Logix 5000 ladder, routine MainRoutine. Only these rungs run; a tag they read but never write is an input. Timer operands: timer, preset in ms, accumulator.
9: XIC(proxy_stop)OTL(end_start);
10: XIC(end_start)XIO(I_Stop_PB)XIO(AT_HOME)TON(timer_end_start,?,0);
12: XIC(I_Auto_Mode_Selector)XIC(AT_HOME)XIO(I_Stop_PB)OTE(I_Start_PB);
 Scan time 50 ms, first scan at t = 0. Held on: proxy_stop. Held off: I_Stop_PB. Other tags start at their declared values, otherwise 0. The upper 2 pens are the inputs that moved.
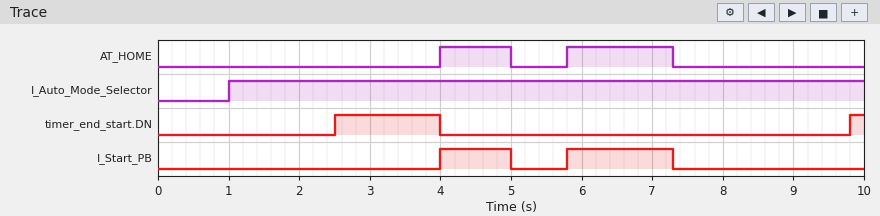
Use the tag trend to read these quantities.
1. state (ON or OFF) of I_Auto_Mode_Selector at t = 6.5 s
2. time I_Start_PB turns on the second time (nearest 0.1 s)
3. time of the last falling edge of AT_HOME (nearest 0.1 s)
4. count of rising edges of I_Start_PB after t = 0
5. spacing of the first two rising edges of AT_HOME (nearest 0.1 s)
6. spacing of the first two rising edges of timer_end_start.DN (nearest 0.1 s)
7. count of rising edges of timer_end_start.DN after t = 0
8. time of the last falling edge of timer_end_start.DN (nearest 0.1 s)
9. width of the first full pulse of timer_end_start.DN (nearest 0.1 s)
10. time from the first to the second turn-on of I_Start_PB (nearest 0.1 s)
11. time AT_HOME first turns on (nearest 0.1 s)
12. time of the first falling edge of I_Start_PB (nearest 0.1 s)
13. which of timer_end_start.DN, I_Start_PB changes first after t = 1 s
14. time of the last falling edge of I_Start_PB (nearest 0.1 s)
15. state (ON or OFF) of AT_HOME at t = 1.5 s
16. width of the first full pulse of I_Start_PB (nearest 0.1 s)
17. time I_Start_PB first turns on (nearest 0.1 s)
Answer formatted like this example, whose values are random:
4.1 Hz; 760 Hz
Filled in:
ON; 5.8 s; 7.3 s; 2; 1.8 s; 7.3 s; 2; 4.0 s; 1.5 s; 1.8 s; 4.0 s; 5.0 s; timer_end_start.DN; 7.3 s; OFF; 1.0 s; 4.0 s
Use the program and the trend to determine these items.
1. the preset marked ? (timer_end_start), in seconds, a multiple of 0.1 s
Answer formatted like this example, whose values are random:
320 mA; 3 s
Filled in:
2.5 s
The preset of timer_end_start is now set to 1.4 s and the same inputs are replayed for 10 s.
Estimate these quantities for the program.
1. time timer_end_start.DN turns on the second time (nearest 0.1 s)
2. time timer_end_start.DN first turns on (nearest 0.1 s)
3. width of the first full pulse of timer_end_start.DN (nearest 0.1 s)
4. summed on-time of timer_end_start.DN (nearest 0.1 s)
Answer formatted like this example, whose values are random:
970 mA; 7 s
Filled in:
8.7 s; 1.4 s; 2.6 s; 3.9 s
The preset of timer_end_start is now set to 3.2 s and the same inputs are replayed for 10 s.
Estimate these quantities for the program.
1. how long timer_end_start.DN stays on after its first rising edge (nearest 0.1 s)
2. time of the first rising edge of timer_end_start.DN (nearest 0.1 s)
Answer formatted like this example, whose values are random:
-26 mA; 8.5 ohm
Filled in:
0.8 s; 3.2 s
